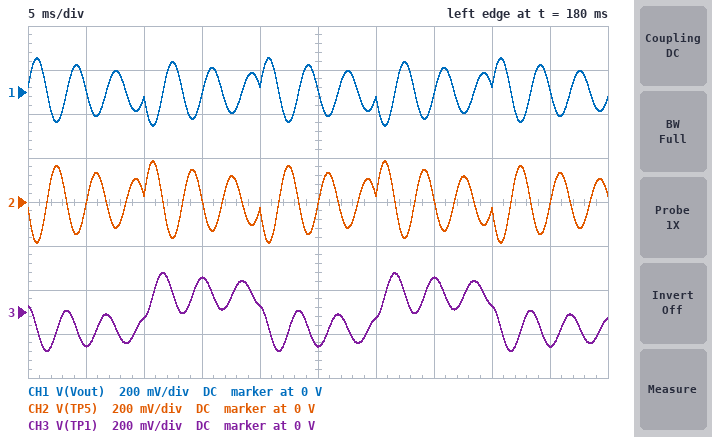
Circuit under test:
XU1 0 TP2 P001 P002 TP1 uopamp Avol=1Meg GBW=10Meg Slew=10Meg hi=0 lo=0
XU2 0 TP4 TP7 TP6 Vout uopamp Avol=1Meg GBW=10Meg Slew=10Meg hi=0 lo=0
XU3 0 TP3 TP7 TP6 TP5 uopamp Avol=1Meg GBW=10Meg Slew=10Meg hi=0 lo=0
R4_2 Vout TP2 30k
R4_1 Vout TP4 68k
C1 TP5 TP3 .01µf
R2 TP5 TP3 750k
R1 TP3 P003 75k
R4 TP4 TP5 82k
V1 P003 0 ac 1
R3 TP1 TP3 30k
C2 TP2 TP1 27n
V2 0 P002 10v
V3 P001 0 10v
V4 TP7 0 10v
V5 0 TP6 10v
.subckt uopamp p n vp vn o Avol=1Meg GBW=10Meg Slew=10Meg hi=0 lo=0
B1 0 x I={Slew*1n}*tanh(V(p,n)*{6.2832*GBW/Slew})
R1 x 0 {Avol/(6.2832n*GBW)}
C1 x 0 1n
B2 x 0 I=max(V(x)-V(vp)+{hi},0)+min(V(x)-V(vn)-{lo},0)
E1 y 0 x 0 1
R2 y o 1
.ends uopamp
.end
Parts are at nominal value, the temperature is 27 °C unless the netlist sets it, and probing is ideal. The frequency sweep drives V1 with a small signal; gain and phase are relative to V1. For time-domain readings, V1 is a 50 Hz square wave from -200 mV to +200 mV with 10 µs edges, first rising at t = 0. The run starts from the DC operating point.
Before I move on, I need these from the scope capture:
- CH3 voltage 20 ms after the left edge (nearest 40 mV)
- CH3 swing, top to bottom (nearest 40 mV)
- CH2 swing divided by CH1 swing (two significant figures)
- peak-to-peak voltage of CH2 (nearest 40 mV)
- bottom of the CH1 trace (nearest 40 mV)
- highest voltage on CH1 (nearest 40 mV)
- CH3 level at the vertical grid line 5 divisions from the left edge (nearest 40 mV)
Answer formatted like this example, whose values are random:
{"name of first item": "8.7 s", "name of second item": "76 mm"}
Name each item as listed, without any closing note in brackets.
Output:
{"CH3 voltage 20 ms after the left edge": "40 mV", "CH3 swing, top to bottom": "360 mV", "CH2 swing divided by CH1 swing": "1.2", "peak-to-peak voltage of CH2": "360 mV", "bottom of the CH1 trace": "-160 mV", "highest voltage on CH1": "160 mV", "CH3 level at the vertical grid line 5 divisions from the left edge": "-160 mV"}
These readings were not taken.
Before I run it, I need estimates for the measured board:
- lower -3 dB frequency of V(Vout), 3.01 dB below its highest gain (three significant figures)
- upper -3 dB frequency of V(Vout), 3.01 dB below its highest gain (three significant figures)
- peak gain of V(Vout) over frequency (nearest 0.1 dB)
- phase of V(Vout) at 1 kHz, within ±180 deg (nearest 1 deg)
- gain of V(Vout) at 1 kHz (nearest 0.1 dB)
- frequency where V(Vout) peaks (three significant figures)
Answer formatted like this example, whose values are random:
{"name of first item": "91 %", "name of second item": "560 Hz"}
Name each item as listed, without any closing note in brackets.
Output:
{"lower -3 dB frequency of V(Vout), 3.01 dB below its highest gain": "284 Hz", "upper -3 dB frequency of V(Vout), 3.01 dB below its highest gain": "305 Hz", "peak gain of V(Vout) over frequency": "18.4 dB", "phase of V(Vout) at 1 kHz, within ±180 deg": "-89 deg", "gain of V(Vout) at 1 kHz": "-14.3 dB", "frequency where V(Vout) peaks": "294 Hz"}
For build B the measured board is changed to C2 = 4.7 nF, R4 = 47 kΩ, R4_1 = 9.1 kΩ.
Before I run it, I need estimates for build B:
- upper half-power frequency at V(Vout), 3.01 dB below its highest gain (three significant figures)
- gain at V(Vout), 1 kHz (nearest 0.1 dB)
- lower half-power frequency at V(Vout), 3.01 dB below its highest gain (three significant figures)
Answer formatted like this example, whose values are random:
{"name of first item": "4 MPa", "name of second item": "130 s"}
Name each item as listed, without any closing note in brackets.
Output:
{"upper half-power frequency at V(Vout), 3.01 dB below its highest gain": "351 Hz", "gain at V(Vout), 1 kHz": "-26.7 dB", "lower half-power frequency at V(Vout), 3.01 dB below its highest gain": "330 Hz"}
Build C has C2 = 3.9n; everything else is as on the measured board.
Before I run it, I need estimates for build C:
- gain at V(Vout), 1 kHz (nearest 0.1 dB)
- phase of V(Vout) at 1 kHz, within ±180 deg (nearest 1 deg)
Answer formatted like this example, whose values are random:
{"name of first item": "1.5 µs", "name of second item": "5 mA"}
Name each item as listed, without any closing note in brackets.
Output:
{"gain at V(Vout), 1 kHz": "-7.2 dB", "phase of V(Vout) at 1 kHz, within ±180 deg": "-87 deg"}
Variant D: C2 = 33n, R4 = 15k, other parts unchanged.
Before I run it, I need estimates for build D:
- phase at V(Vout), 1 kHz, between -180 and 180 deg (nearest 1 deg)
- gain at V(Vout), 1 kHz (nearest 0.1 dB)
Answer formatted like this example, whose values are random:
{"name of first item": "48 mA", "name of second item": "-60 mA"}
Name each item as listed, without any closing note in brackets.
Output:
{"phase at V(Vout), 1 kHz, between -180 and 180 deg": "-88 deg", "gain at V(Vout), 1 kHz": "3.9 dB"}
